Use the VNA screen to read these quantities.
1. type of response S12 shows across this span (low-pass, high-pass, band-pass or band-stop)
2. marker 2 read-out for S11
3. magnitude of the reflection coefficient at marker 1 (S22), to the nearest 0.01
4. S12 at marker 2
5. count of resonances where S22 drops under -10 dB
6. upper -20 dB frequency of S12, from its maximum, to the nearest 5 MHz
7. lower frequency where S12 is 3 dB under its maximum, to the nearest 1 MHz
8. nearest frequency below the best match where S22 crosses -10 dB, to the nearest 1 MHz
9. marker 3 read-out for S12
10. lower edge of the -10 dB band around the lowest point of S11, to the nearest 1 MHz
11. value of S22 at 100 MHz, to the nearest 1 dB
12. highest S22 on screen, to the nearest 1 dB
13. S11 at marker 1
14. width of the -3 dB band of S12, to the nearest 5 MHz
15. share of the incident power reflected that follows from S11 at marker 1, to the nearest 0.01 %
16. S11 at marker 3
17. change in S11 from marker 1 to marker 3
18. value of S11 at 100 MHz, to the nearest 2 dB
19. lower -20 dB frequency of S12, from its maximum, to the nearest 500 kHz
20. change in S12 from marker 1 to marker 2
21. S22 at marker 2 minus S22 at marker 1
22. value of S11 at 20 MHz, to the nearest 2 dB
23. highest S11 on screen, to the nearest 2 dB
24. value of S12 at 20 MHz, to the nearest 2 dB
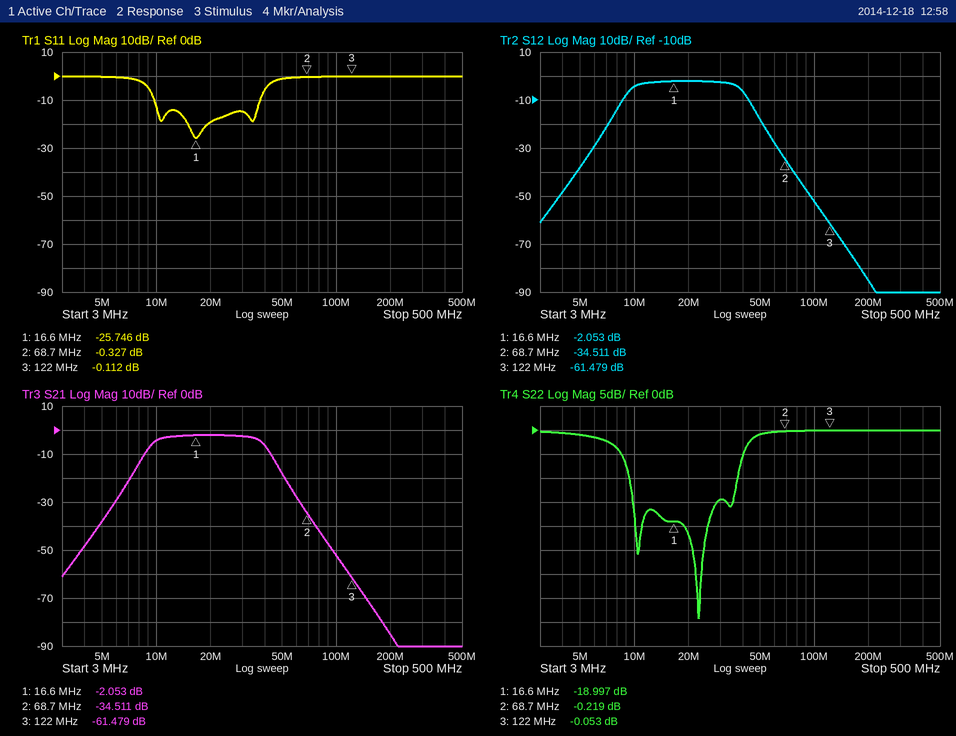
band-pass
-0.327 dB
0.11
-34.511 dB
2
55 MHz
10 MHz
9 MHz
-61.479 dB
10 MHz
0 dB
0 dB
-25.746 dB
30 MHz
0.27 %
-0.112 dB
25.634 dB
0 dB
7.0 MHz
-32.458 dB
18.778 dB
-20 dB
0 dB
-2 dB
